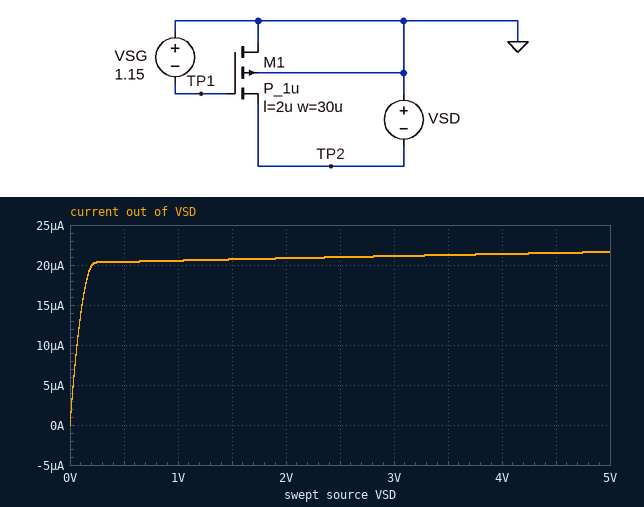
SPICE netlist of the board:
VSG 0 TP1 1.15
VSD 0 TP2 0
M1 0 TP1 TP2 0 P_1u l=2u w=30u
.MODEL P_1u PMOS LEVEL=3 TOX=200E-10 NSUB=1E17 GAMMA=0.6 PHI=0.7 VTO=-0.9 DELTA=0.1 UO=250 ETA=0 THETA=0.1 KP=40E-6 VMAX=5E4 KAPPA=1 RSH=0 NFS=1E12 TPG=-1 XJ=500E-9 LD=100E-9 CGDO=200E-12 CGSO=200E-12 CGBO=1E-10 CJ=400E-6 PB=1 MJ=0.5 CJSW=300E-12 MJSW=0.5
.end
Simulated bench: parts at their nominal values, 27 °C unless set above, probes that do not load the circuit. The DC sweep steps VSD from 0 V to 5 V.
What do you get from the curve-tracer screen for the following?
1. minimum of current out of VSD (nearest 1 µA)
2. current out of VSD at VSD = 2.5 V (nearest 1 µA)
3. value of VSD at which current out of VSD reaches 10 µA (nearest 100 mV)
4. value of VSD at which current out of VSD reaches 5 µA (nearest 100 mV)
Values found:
0 A
21 µA
100 mV
0 V
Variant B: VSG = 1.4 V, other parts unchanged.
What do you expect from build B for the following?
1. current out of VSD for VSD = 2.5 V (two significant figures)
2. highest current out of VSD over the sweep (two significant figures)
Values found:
71 µA
74 µA
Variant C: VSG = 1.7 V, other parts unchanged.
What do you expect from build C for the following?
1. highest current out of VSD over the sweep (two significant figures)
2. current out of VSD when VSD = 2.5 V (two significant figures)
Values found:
170 µA
160 µA
